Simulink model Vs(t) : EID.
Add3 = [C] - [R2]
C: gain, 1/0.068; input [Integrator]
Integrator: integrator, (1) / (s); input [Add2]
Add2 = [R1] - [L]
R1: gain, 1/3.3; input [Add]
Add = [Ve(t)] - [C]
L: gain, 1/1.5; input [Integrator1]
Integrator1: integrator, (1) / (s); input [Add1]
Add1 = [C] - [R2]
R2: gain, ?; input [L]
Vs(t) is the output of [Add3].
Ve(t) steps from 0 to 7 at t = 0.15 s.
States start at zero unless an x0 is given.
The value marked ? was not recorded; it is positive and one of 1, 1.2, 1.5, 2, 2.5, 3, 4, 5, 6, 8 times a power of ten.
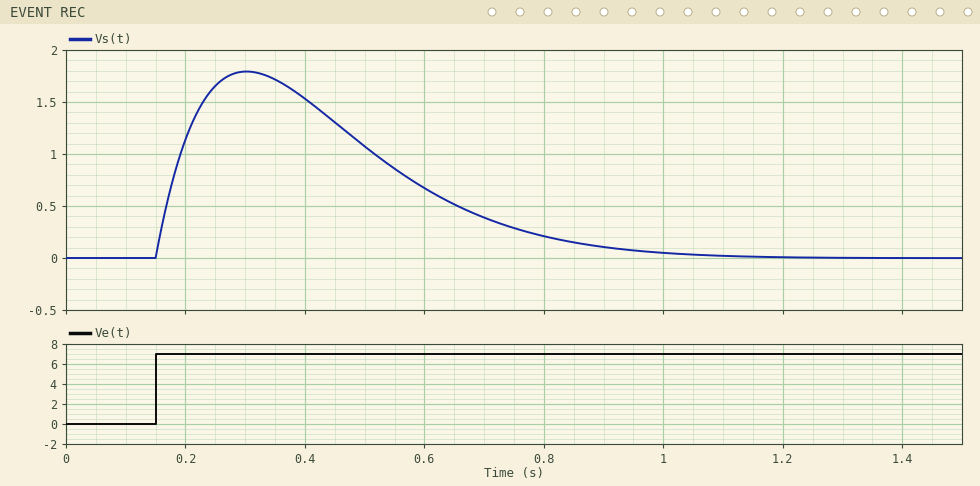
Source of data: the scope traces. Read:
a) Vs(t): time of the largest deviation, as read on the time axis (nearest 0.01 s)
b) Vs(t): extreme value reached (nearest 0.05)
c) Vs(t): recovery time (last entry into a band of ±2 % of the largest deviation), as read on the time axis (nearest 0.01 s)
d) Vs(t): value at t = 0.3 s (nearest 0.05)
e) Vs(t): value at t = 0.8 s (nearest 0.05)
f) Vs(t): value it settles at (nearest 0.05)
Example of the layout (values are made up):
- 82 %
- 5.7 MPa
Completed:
- 0.30 s
- 1.80
- 1.04 s
- 1.80
- 0.20
- 0.00
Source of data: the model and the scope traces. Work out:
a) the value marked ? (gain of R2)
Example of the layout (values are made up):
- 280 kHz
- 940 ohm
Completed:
- 12
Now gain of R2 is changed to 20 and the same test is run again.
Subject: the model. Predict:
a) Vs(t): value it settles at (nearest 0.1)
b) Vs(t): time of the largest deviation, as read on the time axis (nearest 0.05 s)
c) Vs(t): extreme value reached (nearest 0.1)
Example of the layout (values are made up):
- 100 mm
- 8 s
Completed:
- 0.0
- 0.25 s
- 1.3
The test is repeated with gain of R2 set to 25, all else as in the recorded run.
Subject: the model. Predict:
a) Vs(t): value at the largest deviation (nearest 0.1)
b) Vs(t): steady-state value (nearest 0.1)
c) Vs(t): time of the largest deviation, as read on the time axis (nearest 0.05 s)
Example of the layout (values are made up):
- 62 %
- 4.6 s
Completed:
- 1.1
- 0.0
- 0.25 s
